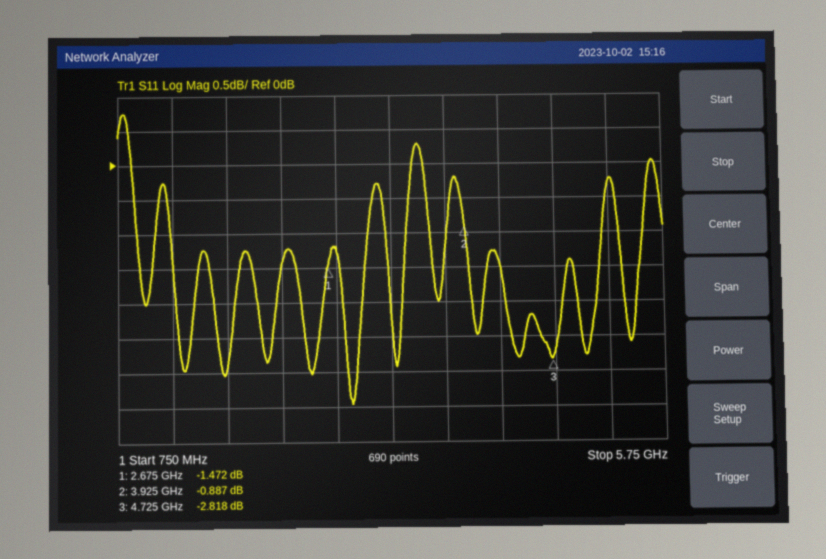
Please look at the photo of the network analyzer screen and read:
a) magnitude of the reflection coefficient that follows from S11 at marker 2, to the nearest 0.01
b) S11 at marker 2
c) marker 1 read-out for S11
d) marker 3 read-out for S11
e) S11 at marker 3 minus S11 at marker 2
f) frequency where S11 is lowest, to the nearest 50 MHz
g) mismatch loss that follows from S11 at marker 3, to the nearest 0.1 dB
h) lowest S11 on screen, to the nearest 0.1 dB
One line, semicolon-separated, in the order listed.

0.90; -0.887 dB; -1.472 dB; -2.818 dB; -1.931 dB; 2.90 GHz; 3.2 dB; -3.5 dB
